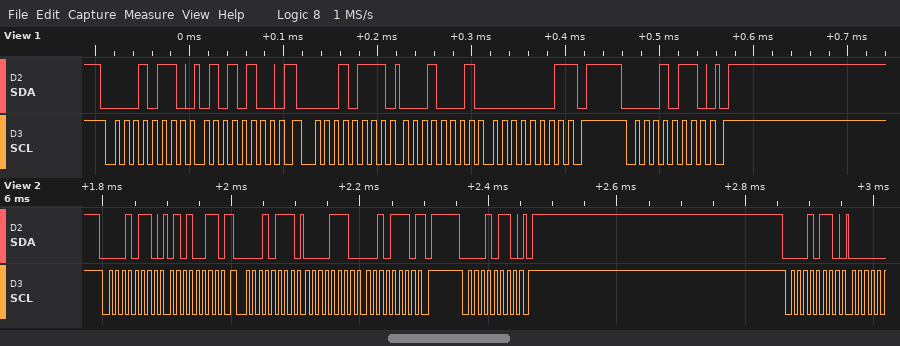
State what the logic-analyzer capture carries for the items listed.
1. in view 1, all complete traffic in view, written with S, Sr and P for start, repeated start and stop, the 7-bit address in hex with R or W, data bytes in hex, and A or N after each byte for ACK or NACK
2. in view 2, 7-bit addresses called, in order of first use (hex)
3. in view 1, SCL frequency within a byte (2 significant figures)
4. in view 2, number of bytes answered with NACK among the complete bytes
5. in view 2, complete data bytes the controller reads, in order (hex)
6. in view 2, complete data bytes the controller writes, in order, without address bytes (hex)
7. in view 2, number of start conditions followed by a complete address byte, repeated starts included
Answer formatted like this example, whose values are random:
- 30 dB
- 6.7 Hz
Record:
- S 0BW A 54 A Sr 0BR A 11 A 01 N P S 0BW A P
- 0x0B
- 100 kHz
- 1
- 0E 2E
- 53
- 4
